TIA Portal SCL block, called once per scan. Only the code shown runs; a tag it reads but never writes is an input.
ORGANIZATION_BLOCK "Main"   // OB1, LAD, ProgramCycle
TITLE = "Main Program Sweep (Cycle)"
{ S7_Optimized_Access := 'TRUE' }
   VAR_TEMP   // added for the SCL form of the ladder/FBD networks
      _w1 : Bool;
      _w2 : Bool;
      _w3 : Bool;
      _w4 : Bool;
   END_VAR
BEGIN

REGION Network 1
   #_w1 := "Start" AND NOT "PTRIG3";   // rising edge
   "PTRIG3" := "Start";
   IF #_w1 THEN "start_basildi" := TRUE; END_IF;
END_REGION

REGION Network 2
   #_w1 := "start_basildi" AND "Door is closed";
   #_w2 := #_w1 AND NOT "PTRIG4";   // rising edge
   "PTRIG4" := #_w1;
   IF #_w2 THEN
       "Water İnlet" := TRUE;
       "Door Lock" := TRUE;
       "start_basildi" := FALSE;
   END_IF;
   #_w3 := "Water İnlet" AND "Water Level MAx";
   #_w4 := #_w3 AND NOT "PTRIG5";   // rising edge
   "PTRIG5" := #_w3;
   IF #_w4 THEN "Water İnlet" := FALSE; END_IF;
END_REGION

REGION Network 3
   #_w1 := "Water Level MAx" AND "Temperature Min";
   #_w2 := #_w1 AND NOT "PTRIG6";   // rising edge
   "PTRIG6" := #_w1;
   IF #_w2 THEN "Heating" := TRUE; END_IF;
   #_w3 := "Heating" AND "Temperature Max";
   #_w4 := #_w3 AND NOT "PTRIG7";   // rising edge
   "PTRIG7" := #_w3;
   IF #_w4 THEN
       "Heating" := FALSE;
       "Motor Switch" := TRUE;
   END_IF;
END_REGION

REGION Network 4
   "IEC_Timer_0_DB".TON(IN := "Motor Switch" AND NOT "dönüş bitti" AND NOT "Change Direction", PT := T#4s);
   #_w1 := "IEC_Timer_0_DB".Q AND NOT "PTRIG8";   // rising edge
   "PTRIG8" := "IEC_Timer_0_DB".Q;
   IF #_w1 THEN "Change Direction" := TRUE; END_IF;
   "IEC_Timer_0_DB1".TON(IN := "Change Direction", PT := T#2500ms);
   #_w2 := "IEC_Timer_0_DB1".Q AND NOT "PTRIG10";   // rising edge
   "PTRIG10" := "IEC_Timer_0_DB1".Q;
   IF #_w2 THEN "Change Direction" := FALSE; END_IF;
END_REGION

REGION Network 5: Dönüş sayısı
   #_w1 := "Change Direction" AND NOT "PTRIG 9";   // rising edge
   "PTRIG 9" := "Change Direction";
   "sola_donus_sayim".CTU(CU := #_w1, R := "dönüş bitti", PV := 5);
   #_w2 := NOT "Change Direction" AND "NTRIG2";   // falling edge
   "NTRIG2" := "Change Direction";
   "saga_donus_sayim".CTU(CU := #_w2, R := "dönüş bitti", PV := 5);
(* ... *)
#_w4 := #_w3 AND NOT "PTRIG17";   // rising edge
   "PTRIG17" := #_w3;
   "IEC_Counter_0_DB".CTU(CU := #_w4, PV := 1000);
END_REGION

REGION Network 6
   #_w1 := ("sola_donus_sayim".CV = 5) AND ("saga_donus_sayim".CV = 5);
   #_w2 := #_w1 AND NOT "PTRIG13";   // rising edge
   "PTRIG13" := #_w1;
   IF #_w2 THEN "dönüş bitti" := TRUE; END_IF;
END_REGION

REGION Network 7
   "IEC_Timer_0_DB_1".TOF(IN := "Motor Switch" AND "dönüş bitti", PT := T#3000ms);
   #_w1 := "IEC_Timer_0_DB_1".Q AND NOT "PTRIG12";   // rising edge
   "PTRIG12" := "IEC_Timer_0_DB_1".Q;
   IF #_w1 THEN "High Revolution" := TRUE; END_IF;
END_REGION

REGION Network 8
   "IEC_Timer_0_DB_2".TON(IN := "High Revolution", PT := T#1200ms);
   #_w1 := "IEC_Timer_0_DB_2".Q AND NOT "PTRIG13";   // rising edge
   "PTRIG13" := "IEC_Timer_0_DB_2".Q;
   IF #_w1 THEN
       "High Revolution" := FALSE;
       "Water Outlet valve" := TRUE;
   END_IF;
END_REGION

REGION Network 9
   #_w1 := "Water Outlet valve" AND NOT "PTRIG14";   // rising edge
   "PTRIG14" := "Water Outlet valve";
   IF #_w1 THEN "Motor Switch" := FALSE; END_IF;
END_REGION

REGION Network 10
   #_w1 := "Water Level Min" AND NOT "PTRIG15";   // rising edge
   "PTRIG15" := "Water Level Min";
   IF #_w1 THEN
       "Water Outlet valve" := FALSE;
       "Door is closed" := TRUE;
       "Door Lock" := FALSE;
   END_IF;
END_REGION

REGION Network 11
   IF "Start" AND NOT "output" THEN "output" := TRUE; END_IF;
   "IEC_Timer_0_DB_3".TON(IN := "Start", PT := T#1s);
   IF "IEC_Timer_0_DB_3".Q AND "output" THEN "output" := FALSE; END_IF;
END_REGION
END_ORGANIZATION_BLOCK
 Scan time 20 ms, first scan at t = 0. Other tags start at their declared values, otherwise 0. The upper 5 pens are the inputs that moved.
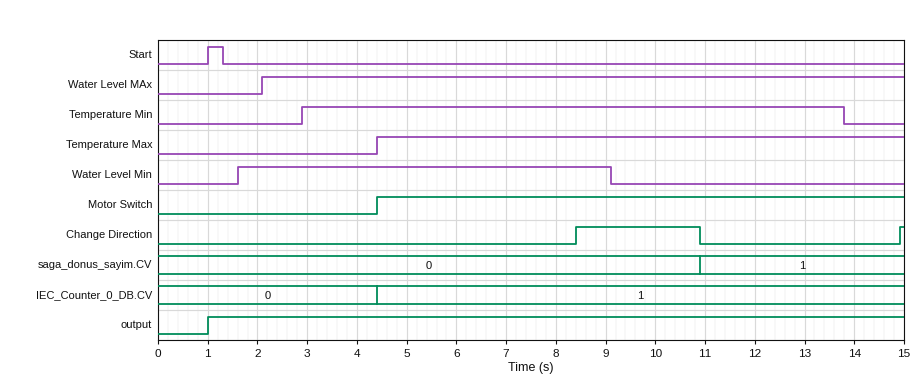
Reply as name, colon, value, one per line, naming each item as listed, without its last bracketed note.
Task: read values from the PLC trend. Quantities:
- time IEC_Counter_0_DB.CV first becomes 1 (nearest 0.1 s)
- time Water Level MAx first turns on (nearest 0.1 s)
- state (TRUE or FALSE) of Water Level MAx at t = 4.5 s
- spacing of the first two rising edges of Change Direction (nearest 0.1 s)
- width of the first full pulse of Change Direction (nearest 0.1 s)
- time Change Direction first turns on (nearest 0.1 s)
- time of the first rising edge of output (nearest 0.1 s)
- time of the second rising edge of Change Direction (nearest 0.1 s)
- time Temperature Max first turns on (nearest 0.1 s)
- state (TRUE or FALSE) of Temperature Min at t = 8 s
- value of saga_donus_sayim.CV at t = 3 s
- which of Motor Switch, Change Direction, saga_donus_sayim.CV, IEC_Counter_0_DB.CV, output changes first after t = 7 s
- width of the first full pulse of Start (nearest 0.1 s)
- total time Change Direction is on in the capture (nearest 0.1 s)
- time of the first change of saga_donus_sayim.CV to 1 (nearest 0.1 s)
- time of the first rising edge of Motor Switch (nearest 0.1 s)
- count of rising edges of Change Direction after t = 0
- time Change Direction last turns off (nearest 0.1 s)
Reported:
time IEC_Counter_0_DB.CV first becomes 1: 4.4 s
time Water Level MAx first turns on: 2.1 s
state (TRUE or FALSE) of Water Level MAx at t = 4.5 s: TRUE
spacing of the first two rising edges of Change Direction: 6.5 s
width of the first full pulse of Change Direction: 2.5 s
time Change Direction first turns on: 8.4 s
time of the first rising edge of output: 1.0 s
time of the second rising edge of Change Direction: 14.9 s
time Temperature Max first turns on: 4.4 s
state (TRUE or FALSE) of Temperature Min at t = 8 s: TRUE
value of saga_donus_sayim.CV at t = 3 s: 0
which of Motor Switch, Change Direction, saga_donus_sayim.CV, IEC_Counter_0_DB.CV, output changes first after t = 7 s: Change Direction
width of the first full pulse of Start: 0.3 s
total time Change Direction is on in the capture: 2.6 s
time of the first change of saga_donus_sayim.CV to 1: 10.9 s
time of the first rising edge of Motor Switch: 4.4 s
count of rising edges of Change Direction after t = 0: 2
time Change Direction last turns off: 10.9 s
